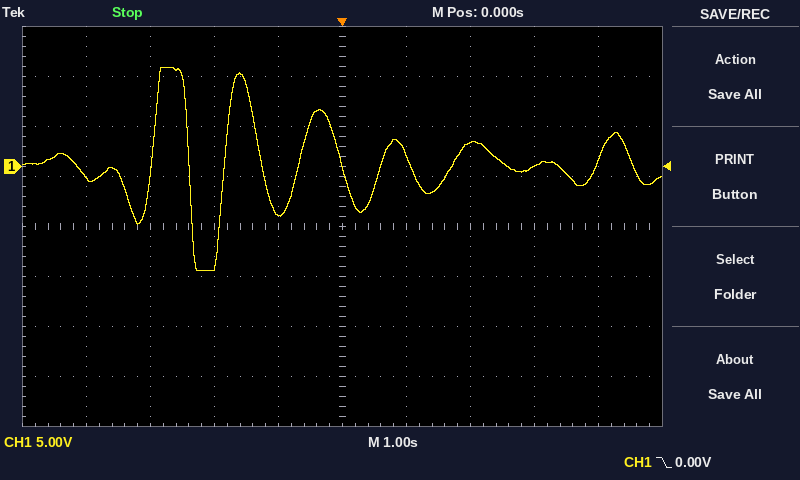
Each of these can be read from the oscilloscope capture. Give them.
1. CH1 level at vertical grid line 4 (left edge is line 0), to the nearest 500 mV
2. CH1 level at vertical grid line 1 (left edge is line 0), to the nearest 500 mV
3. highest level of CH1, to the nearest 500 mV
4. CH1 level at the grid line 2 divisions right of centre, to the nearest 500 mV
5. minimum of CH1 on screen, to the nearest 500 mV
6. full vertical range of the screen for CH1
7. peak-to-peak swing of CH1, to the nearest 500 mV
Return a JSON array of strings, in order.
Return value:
["-5.0 V", "-1.0 V", "10.0 V", "2.5 V", "-10.5 V", "40 V", "20.5 V"]
